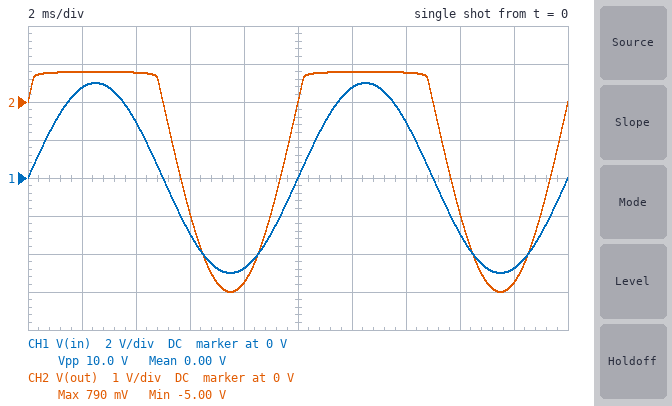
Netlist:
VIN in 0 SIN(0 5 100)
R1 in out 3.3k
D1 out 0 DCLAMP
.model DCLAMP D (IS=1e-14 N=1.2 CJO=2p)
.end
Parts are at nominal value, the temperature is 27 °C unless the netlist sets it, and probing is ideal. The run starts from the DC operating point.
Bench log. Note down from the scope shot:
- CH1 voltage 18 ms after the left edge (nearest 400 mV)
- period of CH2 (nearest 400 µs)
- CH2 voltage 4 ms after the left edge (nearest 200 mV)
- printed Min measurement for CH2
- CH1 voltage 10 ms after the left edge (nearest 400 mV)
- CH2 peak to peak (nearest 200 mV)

-4.8 V
10.0 ms
800 mV
-5.00 V
0 V
5.8 V
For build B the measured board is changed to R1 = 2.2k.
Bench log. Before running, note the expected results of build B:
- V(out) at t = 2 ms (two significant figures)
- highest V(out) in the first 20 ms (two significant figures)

800 mV
810 mV
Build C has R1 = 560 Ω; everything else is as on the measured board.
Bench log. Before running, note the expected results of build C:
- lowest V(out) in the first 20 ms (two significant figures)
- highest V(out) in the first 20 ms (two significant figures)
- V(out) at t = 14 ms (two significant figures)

-5.0 V
850 mV
830 mV
